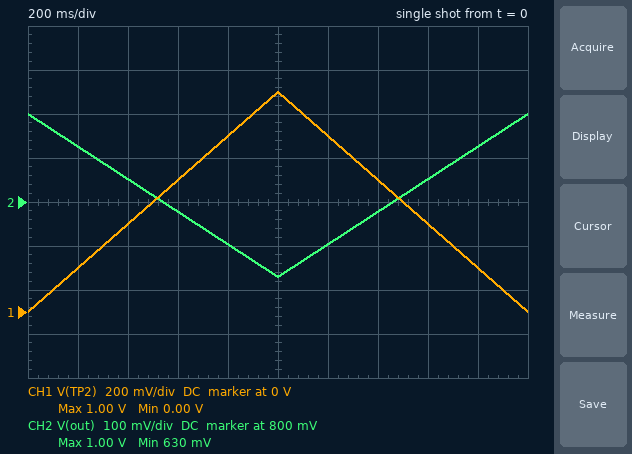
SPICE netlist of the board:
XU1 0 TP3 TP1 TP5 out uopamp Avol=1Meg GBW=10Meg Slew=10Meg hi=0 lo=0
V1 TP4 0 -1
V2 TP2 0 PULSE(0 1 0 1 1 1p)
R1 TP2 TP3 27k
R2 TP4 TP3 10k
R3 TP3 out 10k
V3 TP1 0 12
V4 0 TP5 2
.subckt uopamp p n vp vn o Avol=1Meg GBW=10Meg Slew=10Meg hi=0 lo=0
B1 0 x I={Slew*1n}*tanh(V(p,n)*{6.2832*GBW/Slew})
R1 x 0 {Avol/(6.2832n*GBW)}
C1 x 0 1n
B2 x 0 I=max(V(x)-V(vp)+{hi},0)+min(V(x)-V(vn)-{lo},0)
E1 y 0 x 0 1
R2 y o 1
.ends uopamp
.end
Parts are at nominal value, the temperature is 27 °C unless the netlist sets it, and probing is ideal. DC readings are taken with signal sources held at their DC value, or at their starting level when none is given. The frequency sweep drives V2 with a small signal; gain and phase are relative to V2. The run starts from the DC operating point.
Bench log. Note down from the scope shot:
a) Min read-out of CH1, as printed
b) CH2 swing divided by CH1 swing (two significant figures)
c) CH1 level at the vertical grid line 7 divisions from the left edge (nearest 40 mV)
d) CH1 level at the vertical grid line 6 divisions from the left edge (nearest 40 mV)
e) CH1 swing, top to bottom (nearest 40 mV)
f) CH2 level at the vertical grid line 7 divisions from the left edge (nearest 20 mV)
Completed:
0.00 V
0.37
600 mV
800 mV
1.00 V
780 mV
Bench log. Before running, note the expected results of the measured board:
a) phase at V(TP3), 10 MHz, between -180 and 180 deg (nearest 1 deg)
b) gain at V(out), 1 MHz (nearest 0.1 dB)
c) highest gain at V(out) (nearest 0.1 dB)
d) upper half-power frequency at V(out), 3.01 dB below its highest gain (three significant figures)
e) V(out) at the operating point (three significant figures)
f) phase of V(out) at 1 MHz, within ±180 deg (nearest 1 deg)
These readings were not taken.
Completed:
23 deg
-8.9 dB
-8.6 dB
4.22 MHz
1.00 V
167 deg
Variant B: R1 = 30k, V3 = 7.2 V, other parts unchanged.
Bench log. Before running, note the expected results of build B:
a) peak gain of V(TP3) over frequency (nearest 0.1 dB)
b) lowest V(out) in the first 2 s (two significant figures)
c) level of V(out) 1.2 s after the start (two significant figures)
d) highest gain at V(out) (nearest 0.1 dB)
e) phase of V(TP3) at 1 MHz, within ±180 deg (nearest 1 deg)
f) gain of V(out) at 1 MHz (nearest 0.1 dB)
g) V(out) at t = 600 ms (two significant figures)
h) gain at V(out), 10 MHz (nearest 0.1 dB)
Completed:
-16.9 dB
670 mV
730 mV
-9.5 dB
77 deg
-9.8 dB
800 mV
-17.6 dB
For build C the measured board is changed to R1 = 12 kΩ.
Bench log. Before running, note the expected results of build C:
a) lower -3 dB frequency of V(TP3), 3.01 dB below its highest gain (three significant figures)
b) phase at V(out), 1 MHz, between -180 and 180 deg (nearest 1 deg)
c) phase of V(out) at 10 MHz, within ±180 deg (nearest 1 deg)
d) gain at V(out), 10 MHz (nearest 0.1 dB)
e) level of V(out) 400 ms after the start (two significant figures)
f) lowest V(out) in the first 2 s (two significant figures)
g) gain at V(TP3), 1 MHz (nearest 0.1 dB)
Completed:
3.53 MHz
164 deg
109 deg
-11.1 dB
670 mV
170 mV
-21.9 dB
